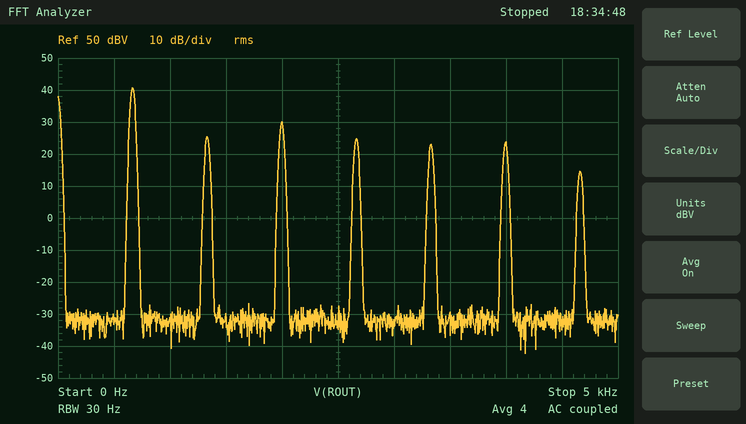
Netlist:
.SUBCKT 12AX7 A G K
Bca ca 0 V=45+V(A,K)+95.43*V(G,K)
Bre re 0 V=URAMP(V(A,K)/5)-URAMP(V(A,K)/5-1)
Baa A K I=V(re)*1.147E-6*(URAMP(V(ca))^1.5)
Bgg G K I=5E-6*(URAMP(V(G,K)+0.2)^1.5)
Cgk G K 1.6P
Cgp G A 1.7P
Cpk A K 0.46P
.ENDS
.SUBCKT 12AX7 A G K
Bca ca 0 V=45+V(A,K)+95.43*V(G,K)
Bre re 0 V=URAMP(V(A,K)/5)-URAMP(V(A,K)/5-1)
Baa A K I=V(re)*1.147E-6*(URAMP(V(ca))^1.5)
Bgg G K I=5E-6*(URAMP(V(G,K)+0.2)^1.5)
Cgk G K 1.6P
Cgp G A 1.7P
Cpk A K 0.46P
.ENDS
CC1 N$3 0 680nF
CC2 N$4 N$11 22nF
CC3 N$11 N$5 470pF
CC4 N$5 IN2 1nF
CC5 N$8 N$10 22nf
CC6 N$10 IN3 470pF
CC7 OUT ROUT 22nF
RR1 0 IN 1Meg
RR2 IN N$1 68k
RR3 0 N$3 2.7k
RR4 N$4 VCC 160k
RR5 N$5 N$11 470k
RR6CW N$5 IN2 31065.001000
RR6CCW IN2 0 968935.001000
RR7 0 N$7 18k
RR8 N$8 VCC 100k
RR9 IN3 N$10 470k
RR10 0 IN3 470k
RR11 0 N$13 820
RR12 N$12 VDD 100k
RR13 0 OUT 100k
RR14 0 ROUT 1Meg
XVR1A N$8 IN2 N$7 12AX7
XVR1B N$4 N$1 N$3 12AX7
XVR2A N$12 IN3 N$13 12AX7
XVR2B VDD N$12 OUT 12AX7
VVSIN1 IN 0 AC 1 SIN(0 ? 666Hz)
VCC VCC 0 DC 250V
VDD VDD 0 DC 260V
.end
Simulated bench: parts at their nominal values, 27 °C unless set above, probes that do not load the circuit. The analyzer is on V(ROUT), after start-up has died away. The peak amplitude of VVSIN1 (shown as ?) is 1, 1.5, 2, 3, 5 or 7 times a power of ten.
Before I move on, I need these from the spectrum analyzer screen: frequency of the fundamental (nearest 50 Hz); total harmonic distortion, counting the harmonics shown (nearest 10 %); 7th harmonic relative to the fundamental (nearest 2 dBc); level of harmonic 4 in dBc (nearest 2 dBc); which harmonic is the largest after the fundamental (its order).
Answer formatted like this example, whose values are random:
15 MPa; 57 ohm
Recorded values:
650 Hz; 40 %; -26 dBc; -16 dBc; 3
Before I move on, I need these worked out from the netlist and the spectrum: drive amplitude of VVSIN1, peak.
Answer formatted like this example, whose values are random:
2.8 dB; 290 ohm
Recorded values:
500 mV
